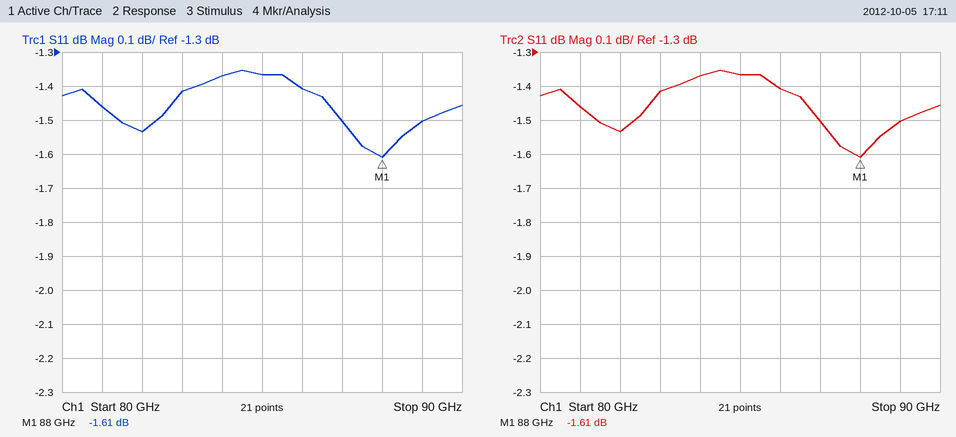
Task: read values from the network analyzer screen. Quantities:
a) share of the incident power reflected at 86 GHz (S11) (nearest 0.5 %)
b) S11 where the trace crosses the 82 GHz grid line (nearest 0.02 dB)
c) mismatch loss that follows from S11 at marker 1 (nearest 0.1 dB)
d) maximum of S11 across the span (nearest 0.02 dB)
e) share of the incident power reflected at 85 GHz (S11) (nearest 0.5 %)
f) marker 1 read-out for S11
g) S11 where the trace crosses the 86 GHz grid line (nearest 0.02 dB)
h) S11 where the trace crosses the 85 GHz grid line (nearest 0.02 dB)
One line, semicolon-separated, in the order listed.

72.5 %; -1.54 dB; 5.1 dB; -1.36 dB; 73.0 %; -1.61 dB; -1.40 dB; -1.36 dB
